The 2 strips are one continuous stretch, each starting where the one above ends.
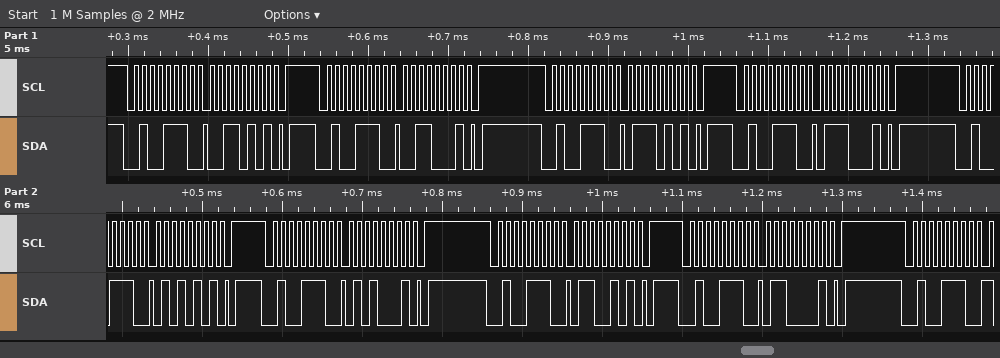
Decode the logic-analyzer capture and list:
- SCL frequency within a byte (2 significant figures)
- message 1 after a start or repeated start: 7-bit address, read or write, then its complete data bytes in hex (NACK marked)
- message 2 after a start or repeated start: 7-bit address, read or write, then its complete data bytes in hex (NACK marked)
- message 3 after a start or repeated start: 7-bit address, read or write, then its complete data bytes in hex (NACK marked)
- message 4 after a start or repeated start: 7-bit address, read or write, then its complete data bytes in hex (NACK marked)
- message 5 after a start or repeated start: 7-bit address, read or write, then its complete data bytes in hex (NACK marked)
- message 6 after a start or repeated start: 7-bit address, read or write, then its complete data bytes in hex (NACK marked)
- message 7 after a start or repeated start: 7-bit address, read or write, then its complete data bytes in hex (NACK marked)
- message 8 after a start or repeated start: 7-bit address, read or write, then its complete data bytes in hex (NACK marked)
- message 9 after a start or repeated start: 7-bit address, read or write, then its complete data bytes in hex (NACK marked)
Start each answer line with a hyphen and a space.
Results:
- 100 kHz
- 0x27 write: 35
- 0x27 write: 31
- 0x27 write: 75
- 0x27 write: 71
- 0x27 write: 55
- 0x27 write: 51
- 0x27 write: 65
- 0x27 write: 61
- 0x27 write
